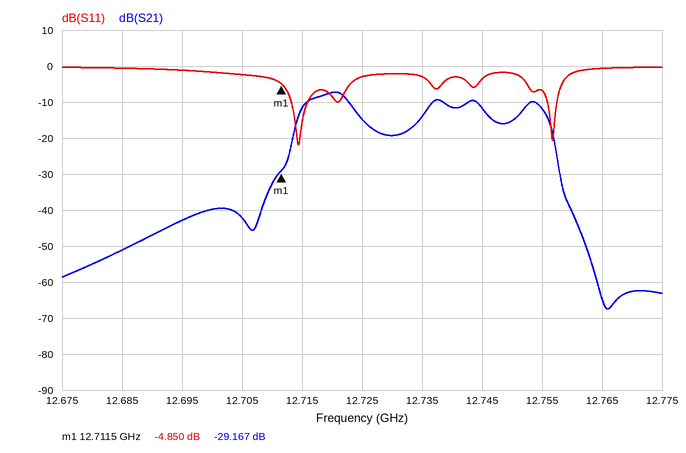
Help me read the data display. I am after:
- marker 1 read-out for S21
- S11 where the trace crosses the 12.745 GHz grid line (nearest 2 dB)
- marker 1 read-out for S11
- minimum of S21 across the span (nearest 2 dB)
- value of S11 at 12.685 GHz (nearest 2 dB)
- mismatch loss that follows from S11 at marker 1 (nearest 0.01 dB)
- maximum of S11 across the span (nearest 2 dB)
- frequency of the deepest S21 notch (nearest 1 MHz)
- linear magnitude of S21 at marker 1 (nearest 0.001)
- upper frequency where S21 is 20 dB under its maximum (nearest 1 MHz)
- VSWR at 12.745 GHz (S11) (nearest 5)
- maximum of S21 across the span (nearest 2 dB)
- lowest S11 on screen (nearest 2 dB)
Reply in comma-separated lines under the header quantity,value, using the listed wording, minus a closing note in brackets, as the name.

quantity,value
marker 1 read-out for S21,-29.167 dB
S11 where the trace crosses the 12.745 GHz grid line,-4 dB
marker 1 read-out for S11,-4.850 dB
minimum of S21 across the span,-68 dB
value of S11 at 12.685 GHz,0 dB
mismatch loss that follows from S11 at marker 1,1.72 dB
maximum of S11 across the span,0 dB
frequency of the deepest S21 notch,12.766 GHz
linear magnitude of S21 at marker 1,0.035
upper frequency where S21 is 20 dB under its maximum,12.758 GHz
VSWR at 12.745 GHz (S11),5
maximum of S21 across the span,-8 dB
lowest S11 on screen,-22 dB
